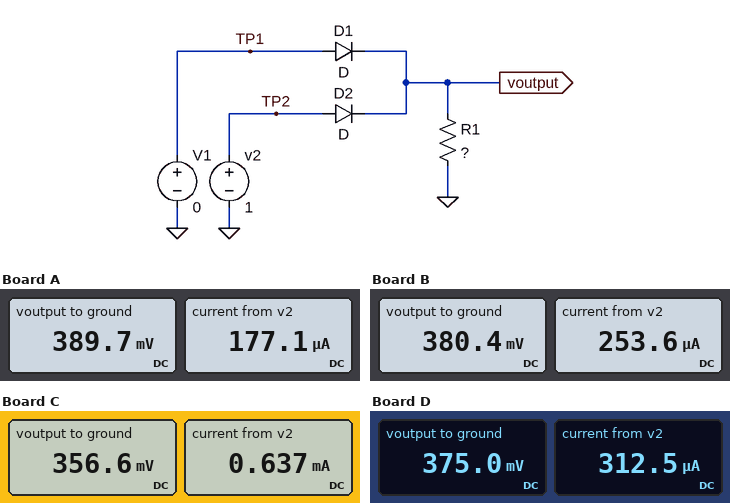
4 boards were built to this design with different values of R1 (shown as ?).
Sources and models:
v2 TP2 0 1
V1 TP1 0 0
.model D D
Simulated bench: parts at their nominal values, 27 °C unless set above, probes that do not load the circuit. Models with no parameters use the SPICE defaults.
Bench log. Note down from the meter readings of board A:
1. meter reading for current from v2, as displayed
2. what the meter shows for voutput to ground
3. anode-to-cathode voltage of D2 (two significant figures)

177.1 µA
389.7 mV
610 mV
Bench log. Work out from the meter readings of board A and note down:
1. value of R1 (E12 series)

2.2 kΩ
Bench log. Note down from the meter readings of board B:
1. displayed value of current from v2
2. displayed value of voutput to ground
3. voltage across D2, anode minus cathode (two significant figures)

253.6 µA
380.4 mV
620 mV
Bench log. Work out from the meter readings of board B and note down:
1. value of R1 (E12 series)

1.5 kΩ
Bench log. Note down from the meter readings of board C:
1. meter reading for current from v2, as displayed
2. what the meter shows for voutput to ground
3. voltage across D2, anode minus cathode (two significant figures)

0.637 mA
356.6 mV
640 mV
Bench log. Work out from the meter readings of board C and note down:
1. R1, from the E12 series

560 Ω
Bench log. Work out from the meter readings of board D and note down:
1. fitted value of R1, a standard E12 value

1.2 kΩ
